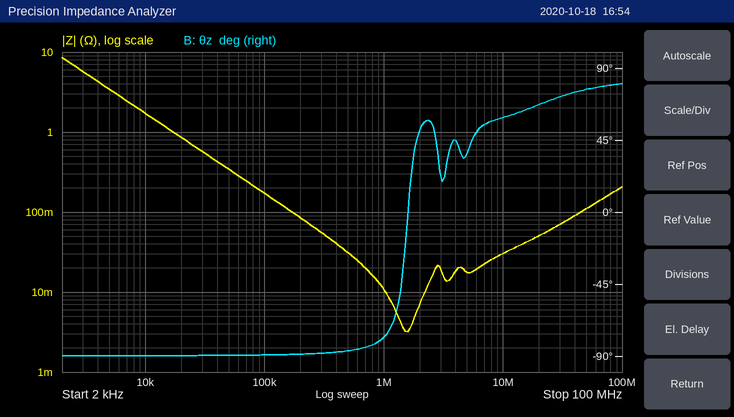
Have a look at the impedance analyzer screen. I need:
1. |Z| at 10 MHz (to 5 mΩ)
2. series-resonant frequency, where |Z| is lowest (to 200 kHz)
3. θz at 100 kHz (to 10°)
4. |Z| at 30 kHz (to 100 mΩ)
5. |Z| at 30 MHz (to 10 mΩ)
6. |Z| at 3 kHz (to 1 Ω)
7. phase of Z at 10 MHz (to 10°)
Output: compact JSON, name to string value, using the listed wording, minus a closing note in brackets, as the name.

{"|Z| at 10 MHz": "30 mΩ", "series-resonant frequency, where |Z| is lowest": "1.6 MHz", "θz at 100 kHz": "-90°", "|Z| at 30 kHz": "600 mΩ", "|Z| at 30 MHz": "70 mΩ", "|Z| at 3 kHz": "6 Ω", "phase of Z at 10 MHz": "60°"}
